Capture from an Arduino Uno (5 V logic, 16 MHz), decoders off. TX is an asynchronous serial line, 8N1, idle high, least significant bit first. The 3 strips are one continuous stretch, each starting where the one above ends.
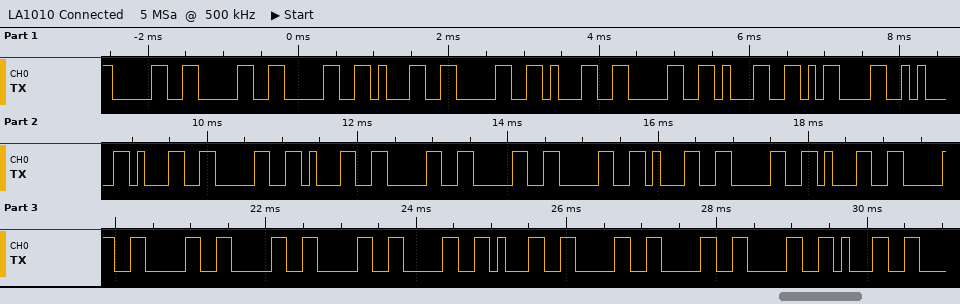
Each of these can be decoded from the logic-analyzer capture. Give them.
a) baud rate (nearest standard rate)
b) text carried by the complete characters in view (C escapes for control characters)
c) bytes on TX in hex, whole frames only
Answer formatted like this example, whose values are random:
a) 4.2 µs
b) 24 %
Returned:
a) 9600 baud
b) "00010101\r\n1010001010000010001"
c) 30 30 30 31 30 31 30 31 0D 0A 31 30 31 30 30 30 31 30 31 30 30 30 30 30 31 30 30 30 31
